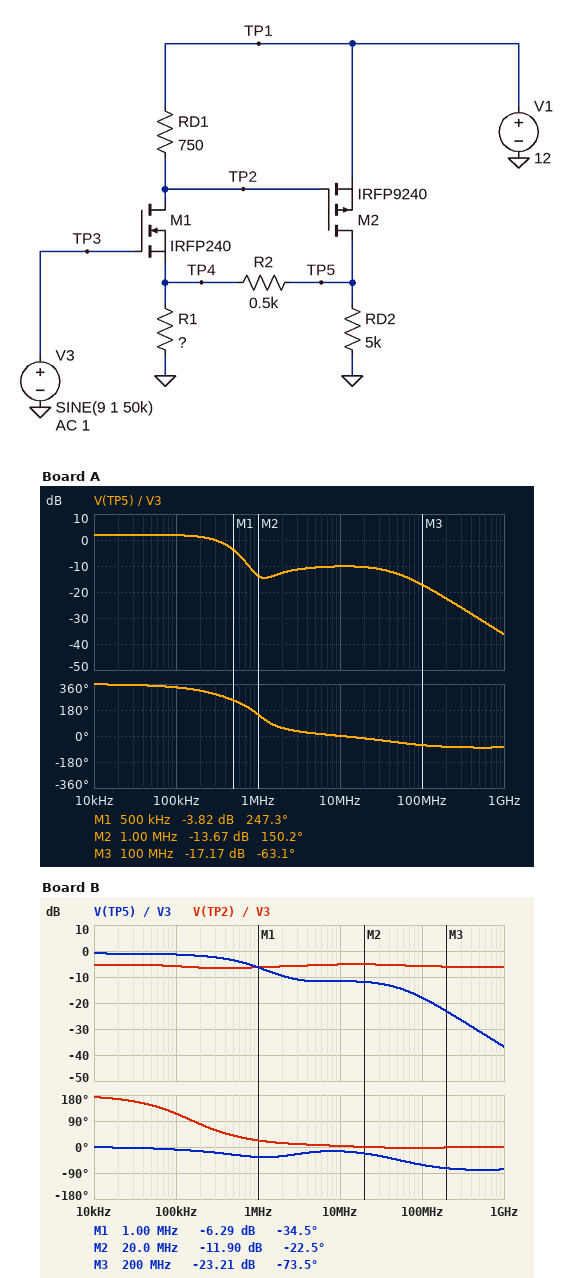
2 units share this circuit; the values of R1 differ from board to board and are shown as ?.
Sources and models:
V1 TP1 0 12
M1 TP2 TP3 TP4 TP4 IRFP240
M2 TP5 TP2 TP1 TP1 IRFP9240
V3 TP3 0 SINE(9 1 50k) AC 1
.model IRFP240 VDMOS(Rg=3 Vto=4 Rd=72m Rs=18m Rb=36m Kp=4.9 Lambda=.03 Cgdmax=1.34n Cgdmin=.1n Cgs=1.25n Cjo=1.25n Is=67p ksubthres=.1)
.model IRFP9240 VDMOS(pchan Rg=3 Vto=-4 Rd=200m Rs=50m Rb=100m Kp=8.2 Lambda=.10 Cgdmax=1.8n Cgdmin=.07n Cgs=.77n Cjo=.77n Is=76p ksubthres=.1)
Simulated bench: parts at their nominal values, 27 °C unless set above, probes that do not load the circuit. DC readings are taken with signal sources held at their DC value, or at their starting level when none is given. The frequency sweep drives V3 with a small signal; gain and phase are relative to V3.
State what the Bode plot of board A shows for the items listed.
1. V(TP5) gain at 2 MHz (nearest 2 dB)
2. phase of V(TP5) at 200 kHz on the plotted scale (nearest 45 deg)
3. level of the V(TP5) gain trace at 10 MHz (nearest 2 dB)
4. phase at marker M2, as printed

-12 dB
315 deg
-10 dB
150.2 deg
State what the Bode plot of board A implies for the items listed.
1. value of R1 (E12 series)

1.2 kΩ
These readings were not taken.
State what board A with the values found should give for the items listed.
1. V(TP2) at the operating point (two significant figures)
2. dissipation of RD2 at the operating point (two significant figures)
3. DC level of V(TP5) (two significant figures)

8.3 V
4.4 mW
4.7 V
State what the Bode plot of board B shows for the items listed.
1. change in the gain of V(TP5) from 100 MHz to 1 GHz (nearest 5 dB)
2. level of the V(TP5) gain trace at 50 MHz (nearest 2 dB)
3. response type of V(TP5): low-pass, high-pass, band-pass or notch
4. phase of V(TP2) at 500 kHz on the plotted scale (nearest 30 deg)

-20 dB
-14 dB
low-pass
30 deg
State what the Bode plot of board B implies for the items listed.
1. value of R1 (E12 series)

1.8 kΩ
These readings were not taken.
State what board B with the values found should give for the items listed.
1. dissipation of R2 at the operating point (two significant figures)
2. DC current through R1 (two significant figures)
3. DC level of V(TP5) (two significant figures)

430 µW
2.8 mA
4.6 V
